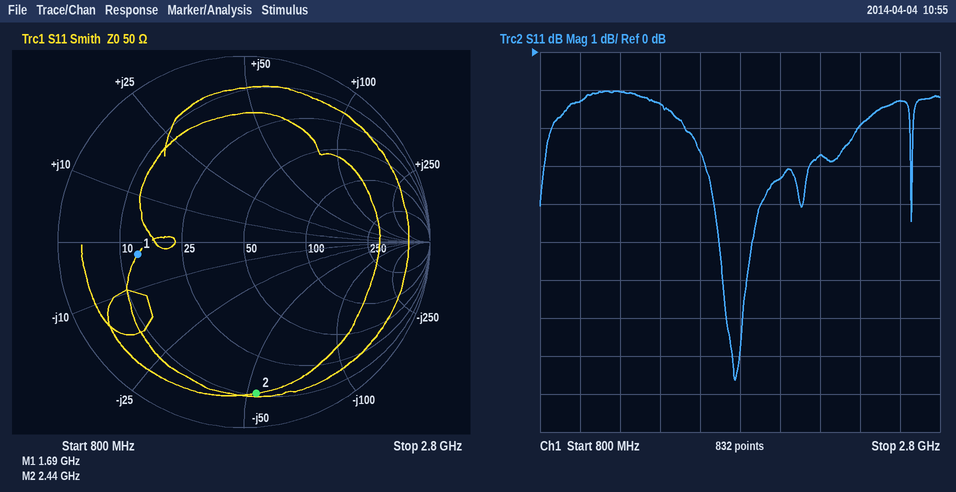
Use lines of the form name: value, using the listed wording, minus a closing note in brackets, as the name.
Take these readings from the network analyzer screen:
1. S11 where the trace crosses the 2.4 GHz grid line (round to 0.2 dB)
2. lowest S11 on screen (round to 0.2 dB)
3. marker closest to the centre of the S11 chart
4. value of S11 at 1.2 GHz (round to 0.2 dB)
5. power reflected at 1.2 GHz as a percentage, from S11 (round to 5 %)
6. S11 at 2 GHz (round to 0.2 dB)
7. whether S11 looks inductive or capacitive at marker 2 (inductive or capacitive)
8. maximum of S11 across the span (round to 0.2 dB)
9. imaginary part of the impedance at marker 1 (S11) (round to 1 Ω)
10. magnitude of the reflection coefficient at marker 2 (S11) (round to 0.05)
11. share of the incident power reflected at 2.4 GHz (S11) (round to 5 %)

S11 where the trace crosses the 2.4 GHz grid line: -2.0 dB
lowest S11 on screen: -8.6 dB
marker closest to the centre of the S11 chart: marker 1
value of S11 at 1.2 GHz: -1.0 dB
power reflected at 1.2 GHz as a percentage, from S11: 80 %
S11 at 2 GHz: -3.4 dB
whether S11 looks inductive or capacitive at marker 2: capacitive
maximum of S11 across the span: -1.0 dB
imaginary part of the impedance at marker 1 (S11): -3 Ω
magnitude of the reflection coefficient at marker 2 (S11): 0.80
share of the incident power reflected at 2.4 GHz (S11): 65 %
